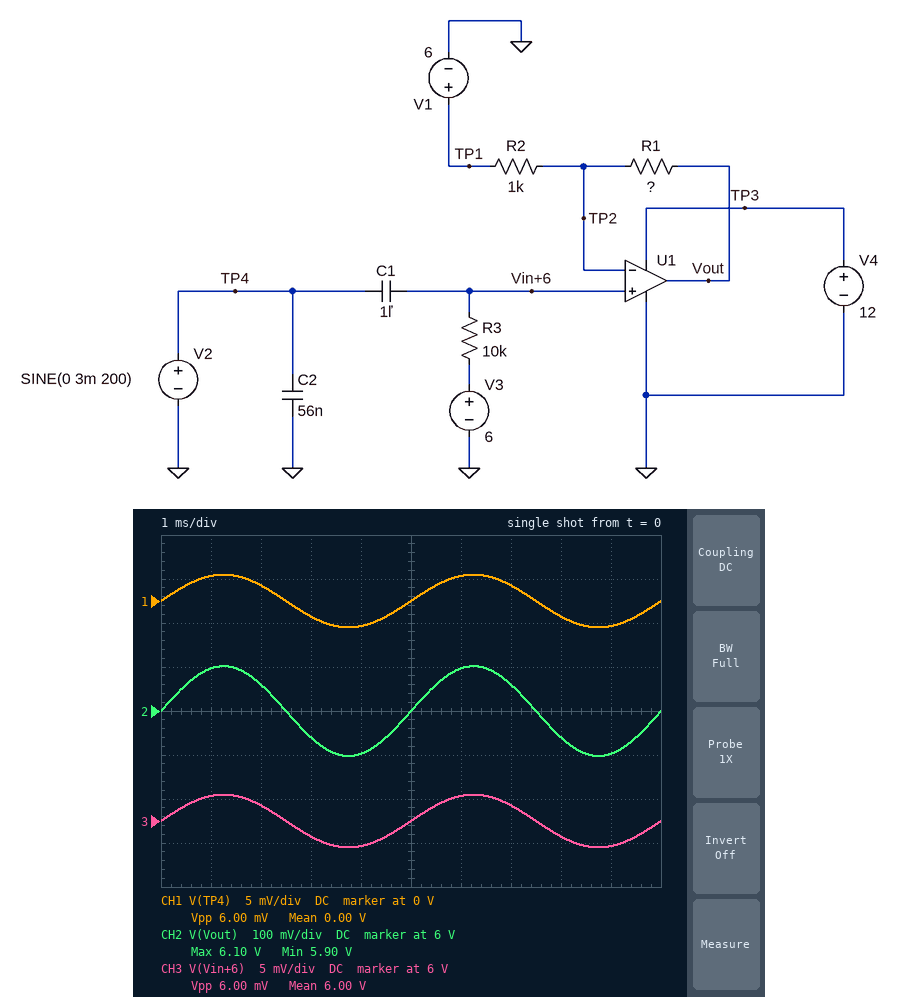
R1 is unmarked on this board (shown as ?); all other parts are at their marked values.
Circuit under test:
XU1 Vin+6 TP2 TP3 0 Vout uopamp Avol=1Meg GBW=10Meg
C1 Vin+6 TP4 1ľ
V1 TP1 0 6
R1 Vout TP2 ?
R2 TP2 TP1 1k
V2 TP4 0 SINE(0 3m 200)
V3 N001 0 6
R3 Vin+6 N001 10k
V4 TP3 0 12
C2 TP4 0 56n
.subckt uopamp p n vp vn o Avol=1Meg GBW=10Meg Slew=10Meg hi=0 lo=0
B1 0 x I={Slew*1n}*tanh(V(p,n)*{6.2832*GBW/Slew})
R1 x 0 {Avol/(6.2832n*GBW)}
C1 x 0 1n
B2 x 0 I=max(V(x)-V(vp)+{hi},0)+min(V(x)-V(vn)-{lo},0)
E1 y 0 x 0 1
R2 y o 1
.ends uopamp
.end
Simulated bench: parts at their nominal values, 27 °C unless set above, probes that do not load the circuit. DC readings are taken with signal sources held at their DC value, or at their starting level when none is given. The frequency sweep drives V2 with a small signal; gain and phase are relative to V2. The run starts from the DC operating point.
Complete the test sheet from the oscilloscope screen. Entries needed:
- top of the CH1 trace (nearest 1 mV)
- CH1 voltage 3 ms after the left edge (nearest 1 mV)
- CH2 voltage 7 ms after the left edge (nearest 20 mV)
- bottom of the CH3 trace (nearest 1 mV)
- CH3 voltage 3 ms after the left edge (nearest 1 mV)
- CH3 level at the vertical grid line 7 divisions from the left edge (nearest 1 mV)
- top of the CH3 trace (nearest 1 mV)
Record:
3 mV
-2 mV
6.06 V
5.997 V
5.998 V
6.002 V
6.003 V
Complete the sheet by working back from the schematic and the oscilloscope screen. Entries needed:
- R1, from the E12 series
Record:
33 kΩ
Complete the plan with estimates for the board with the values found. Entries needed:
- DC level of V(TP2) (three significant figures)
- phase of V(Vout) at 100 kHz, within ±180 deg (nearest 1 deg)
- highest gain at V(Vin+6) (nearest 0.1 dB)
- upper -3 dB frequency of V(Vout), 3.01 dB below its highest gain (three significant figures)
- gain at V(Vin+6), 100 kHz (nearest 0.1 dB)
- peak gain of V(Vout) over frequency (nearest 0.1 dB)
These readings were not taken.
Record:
6.00 V
-19 deg
0 dB
294 kHz
0 dB
30.6 dB
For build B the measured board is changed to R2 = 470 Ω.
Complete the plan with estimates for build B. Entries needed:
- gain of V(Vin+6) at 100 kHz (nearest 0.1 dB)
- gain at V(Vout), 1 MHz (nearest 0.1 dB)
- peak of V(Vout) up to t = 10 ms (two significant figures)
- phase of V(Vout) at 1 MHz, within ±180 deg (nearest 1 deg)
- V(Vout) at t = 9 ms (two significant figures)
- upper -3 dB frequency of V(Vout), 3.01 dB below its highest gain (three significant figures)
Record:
0 dB
19.9 dB
6.2 V
-82 deg
5.8 V
140 kHz
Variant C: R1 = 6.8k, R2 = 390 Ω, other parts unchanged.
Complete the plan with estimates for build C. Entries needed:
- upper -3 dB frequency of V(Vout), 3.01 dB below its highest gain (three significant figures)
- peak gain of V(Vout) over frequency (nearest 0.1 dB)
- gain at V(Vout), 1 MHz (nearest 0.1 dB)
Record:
542 kHz
25.3 dB
18.9 dB
